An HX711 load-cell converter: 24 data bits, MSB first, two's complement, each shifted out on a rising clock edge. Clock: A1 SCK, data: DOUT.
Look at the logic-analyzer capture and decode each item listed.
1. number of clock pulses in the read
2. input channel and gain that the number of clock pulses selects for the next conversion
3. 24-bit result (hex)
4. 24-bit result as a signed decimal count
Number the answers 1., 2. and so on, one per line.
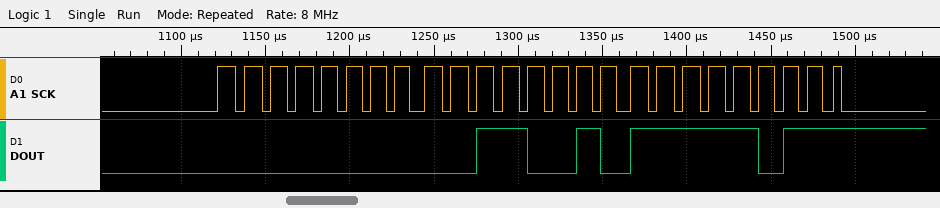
1. 25
2. channel A, gain 128
3. 0x0032FB
4. 13051
